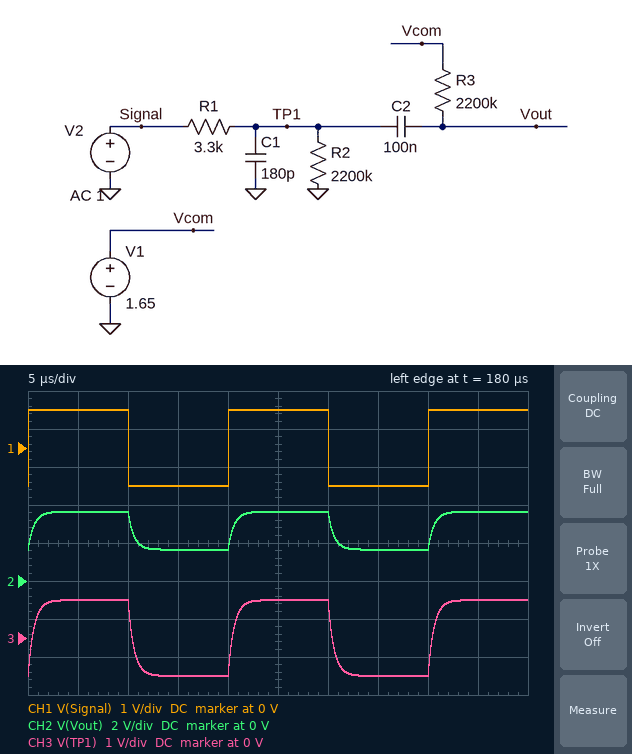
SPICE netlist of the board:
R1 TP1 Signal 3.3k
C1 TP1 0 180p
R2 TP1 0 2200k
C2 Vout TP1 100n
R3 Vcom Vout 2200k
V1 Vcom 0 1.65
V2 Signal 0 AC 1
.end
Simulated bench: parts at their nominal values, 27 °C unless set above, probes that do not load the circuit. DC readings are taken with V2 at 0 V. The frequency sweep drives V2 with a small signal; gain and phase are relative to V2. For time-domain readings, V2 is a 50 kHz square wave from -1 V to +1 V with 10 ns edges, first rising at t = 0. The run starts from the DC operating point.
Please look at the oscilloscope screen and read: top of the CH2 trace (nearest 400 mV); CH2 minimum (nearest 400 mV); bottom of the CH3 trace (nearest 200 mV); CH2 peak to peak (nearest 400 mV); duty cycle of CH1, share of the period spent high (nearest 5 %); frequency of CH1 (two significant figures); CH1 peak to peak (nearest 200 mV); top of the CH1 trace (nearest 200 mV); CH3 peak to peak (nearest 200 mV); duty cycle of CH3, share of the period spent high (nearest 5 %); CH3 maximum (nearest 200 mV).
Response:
3.6 V
1.6 V
-1.0 V
2.0 V
50 %
50 kHz
2.0 V
1.0 V
2.0 V
50 %
1.0 V
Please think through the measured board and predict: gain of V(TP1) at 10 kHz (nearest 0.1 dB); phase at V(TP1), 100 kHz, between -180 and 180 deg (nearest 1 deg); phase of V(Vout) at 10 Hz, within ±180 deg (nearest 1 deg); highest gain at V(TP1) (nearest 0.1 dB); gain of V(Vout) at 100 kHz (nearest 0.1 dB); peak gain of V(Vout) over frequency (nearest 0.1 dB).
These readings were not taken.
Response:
0 dB
-20 deg
4 deg
0 dB
-0.6 dB
0 dB
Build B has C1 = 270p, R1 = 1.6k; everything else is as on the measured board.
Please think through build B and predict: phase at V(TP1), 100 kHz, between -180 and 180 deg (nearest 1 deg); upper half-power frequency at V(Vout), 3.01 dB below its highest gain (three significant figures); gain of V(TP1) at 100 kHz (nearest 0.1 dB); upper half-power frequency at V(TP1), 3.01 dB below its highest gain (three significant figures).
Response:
-15 deg
369 kHz
-0.3 dB
368 kHz
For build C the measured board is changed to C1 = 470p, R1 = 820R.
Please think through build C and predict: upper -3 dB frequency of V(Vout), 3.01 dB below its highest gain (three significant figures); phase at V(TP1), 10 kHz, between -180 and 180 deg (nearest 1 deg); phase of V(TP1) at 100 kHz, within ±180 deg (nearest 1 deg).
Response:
413 kHz
-1 deg
-14 deg
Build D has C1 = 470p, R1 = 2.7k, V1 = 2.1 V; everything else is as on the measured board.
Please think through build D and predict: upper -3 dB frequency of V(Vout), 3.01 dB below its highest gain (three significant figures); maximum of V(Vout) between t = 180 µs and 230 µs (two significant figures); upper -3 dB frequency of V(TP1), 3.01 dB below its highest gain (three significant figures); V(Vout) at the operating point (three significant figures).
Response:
126 kHz
4.1 V
125 kHz
2.10 V
